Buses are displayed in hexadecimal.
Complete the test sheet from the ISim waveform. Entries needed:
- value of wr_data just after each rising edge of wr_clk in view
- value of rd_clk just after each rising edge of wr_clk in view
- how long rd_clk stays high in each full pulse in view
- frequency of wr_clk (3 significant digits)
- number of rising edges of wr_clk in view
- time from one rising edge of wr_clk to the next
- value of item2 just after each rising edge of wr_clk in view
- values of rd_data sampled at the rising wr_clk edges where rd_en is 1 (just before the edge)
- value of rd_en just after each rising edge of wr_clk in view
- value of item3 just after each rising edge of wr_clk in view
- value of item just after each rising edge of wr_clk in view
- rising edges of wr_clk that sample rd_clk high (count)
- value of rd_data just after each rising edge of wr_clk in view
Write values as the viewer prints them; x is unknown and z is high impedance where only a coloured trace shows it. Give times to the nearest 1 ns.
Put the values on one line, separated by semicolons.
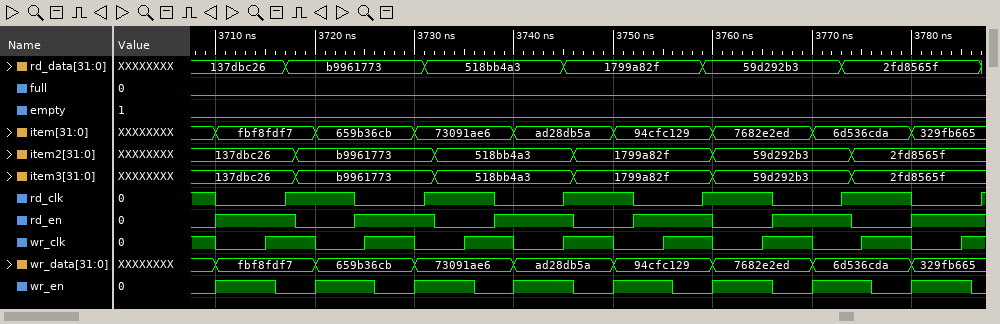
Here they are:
fbf8fdf7, 659b36cb, 73091ae6, ad28db5a, 94cfc129, 7682e2ed, 6d536cda, 329fb665; 0 0 1 1 0 1 1 0; 7 ns, 7 ns, 7 ns, 7 ns, 7 ns; 100 MHz; 8; 10 ns; 137dbc26, b9961773, 518bb4a3, 518bb4a3, 1799a82f, 59d292b3, 2fd8565f, 2fd8565f; 137dbc26, b9961773, 518bb4a3, 1799a82f, 2fd8565f; 1 1 0 1 1 0 0 1; 137dbc26, b9961773, 518bb4a3, 518bb4a3, 1799a82f, 59d292b3, 2fd8565f, 2fd8565f; fbf8fdf7, 659b36cb, 73091ae6, ad28db5a, 94cfc129, 7682e2ed, 6d536cda, 329fb665; 3; 137dbc26, b9961773, 518bb4a3, 1799a82f, 1799a82f, 59d292b3, 2fd8565f, 2fd8565f
